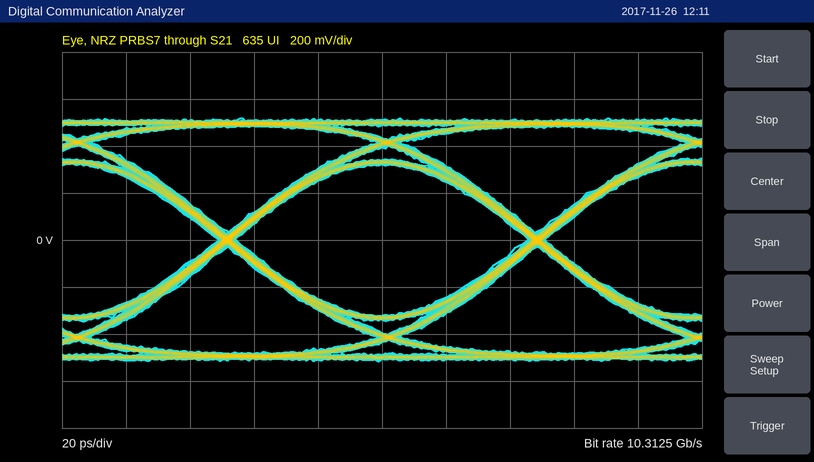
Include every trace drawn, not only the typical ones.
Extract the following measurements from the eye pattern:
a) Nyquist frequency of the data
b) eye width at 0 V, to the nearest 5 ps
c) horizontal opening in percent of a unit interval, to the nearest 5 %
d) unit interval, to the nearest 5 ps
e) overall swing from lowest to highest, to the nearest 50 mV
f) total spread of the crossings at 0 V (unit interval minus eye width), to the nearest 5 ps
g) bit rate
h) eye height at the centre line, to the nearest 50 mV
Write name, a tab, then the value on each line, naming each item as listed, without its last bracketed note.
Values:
Nyquist frequency of the data	5.15625 GHz
eye width at 0 V, to the nearest 5 ps	90 ps
horizontal opening in percent of a unit interval, to the nearest 5 %	95 %
unit interval, to the nearest 5 ps	95 ps
overall swing from lowest to highest, to the nearest 50 mV	1.05 V
total spread of the crossings at 0 V (unit interval minus eye width), to the nearest 5 ps	5 ps
bit rate	10.3125 Gb/s
eye height at the centre line, to the nearest 50 mV	650 mV
